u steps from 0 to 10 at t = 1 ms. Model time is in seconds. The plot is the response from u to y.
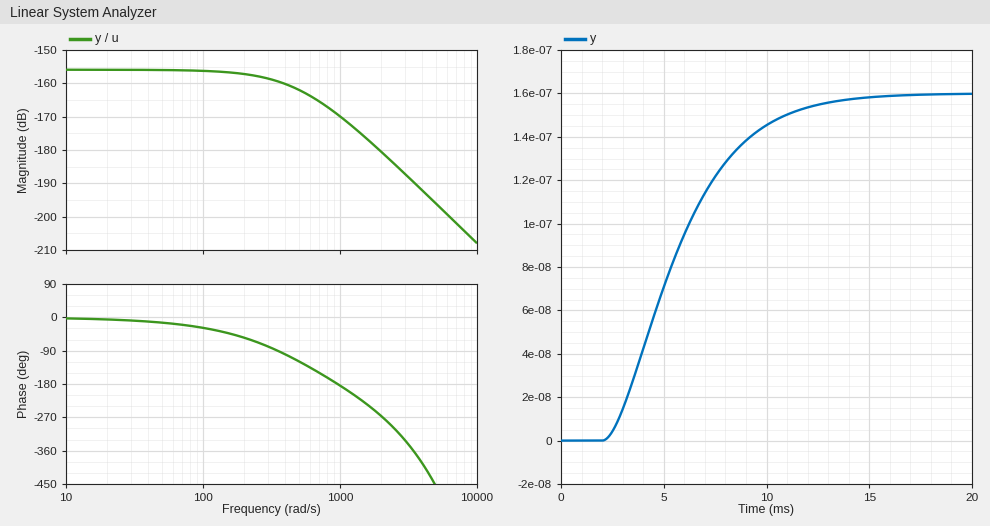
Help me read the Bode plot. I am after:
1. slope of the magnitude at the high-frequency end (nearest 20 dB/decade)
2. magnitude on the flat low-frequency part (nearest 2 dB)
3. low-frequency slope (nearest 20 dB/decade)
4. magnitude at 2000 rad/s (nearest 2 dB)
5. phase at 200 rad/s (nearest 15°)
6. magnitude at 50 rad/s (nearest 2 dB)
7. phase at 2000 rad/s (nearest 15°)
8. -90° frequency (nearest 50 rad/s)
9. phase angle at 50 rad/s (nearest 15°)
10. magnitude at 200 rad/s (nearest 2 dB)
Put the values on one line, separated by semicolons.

-40 dB/decade; -156 dB; 0 dB/decade; -180 dB; -60°; -156 dB; -270°; 350 rad/s; -15°; -158 dB
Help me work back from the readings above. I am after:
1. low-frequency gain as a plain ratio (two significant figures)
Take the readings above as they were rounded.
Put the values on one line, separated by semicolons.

0.000000016
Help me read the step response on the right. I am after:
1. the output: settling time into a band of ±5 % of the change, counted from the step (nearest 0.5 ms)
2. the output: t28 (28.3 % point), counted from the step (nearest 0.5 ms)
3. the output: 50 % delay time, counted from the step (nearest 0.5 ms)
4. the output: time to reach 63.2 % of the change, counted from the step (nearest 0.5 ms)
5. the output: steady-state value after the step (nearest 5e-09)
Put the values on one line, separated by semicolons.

10.5 ms; 3.0 ms; 4.5 ms; 5.5 ms; 0.000000160
